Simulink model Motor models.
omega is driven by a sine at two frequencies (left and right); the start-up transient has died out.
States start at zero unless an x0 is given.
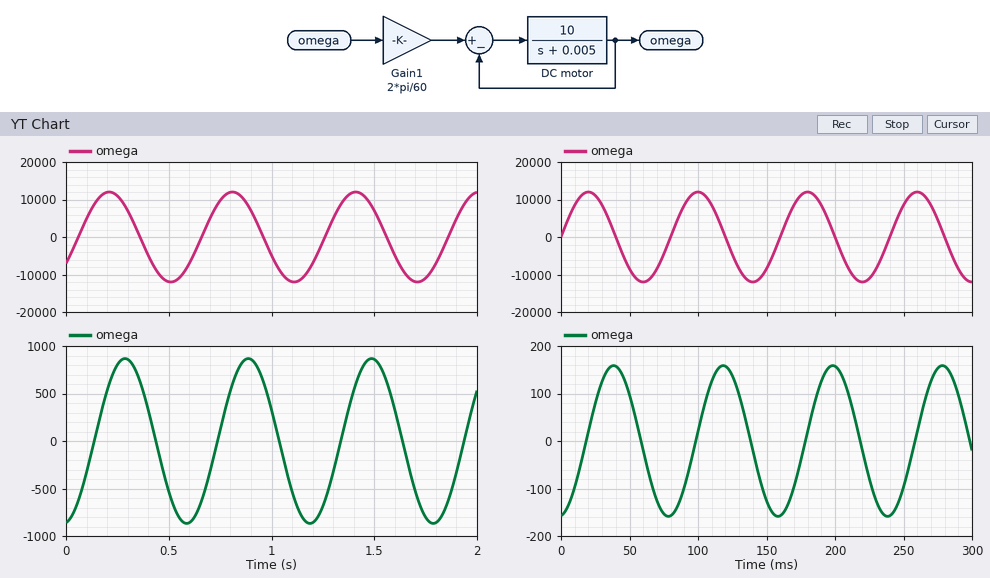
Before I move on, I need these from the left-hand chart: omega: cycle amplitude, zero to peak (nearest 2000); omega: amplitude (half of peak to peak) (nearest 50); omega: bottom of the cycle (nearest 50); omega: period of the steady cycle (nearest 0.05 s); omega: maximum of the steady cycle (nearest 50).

12000
850
-850
0.60 s
850
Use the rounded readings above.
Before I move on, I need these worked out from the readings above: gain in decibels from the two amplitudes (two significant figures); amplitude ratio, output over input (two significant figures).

-23 dB
0.071
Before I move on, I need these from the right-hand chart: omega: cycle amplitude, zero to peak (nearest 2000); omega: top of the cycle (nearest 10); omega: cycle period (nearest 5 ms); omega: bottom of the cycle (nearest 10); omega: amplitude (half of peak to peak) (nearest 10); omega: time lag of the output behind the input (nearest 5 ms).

12000
160
80 ms
-160
160
20 ms
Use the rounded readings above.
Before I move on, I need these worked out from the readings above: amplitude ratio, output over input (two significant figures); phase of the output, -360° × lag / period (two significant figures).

0.013
-90°
